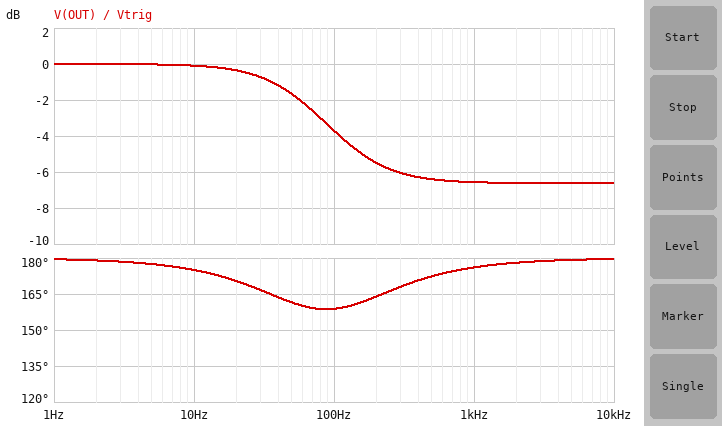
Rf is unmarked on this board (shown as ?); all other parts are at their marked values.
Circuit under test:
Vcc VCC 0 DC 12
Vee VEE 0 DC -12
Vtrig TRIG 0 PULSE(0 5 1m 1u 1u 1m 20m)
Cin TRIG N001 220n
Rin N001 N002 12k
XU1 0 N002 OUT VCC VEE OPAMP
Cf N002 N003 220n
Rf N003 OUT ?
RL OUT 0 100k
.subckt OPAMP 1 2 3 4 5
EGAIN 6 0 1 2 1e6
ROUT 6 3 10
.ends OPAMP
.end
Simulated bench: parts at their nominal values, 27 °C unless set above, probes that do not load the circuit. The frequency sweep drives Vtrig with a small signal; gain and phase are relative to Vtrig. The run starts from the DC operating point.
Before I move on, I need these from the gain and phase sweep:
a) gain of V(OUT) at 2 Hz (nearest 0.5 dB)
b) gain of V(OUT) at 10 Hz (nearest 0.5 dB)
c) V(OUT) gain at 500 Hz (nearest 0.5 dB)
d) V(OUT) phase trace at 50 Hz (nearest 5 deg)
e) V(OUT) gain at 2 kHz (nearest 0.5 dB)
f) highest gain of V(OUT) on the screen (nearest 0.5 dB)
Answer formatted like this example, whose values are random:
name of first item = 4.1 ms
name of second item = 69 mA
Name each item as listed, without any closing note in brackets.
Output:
gain of V(OUT) at 2 Hz = 0 dB
gain of V(OUT) at 10 Hz = 0 dB
V(OUT) gain at 500 Hz = -6.5 dB
V(OUT) phase trace at 50 Hz = 160 deg
V(OUT) gain at 2 kHz = -6.5 dB
highest gain of V(OUT) on the screen = 0 dB
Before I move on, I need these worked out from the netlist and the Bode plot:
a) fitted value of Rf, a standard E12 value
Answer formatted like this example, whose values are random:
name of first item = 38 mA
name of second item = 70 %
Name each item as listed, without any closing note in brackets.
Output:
fitted value of Rf, a standard E12 value = 5.6 kΩ
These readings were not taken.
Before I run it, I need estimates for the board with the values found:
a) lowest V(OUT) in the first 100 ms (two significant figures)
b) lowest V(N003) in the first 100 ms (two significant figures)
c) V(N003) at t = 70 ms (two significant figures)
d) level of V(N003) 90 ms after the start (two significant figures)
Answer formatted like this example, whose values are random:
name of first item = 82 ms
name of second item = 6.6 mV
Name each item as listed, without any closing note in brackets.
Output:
lowest V(OUT) in the first 100 ms = -3.2 V
lowest V(N003) in the first 100 ms = -1.6 V
V(N003) at t = 70 ms = -76 mV
level of V(N003) 90 ms after the start = -76 mV
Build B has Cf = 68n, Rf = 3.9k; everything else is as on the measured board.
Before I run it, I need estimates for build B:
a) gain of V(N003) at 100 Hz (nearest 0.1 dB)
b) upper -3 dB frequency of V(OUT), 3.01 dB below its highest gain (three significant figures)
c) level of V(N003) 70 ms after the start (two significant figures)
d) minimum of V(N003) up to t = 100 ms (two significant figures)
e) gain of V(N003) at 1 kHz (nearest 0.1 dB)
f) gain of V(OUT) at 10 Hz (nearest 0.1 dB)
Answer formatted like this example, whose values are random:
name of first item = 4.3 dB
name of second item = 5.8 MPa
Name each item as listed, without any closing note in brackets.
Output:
gain of V(N003) at 100 Hz = 4.5 dB
upper -3 dB frequency of V(OUT), 3.01 dB below its highest gain = 60.9 Hz
level of V(N003) 70 ms after the start = -250 mV
minimum of V(N003) up to t = 100 ms = -5.1 V
gain of V(N003) at 1 kHz = -14.2 dB
gain of V(OUT) at 10 Hz = 10.1 dB
